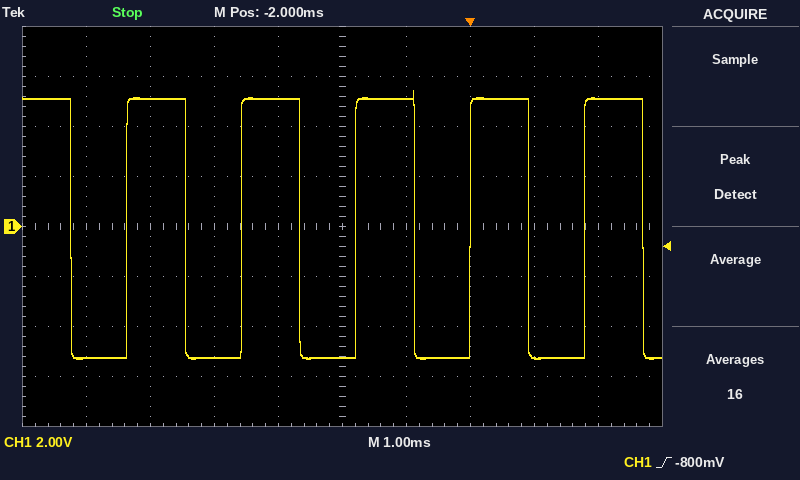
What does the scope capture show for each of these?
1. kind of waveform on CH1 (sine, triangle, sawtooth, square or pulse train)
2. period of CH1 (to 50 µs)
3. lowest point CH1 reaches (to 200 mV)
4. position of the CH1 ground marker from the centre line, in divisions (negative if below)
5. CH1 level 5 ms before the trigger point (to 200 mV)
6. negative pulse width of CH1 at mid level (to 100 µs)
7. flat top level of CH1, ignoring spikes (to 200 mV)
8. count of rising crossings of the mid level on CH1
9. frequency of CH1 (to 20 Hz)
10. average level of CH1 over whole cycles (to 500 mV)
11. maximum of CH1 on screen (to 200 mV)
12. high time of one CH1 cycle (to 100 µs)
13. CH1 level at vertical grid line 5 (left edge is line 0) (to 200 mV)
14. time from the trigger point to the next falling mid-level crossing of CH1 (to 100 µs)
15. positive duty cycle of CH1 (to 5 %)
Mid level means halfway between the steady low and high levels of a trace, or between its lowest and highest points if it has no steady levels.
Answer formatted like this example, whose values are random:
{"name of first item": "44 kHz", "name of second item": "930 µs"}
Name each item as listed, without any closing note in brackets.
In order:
{"kind of waveform on CH1": "square", "period of CH1": "1.80 ms", "lowest point CH1 reaches": "-5.2 V", "position of the CH1 ground marker from the centre line, in divisions": "0.0 div", "CH1 level 5 ms before the trigger point": "5.2 V", "negative pulse width of CH1 at mid level": "900 µs", "flat top level of CH1, ignoring spikes": "5.2 V", "count of rising crossings of the mid level on CH1": "5", "frequency of CH1": "560 Hz", "average level of CH1 over whole cycles": "0.0 V", "maximum of CH1 on screen": "5.4 V", "high time of one CH1 cycle": "900 µs", "CH1 level at vertical grid line 5 (left edge is line 0)": "-5.2 V", "time from the trigger point to the next falling mid-level crossing of CH1": "900 µs", "positive duty cycle of CH1": "50 %"}
